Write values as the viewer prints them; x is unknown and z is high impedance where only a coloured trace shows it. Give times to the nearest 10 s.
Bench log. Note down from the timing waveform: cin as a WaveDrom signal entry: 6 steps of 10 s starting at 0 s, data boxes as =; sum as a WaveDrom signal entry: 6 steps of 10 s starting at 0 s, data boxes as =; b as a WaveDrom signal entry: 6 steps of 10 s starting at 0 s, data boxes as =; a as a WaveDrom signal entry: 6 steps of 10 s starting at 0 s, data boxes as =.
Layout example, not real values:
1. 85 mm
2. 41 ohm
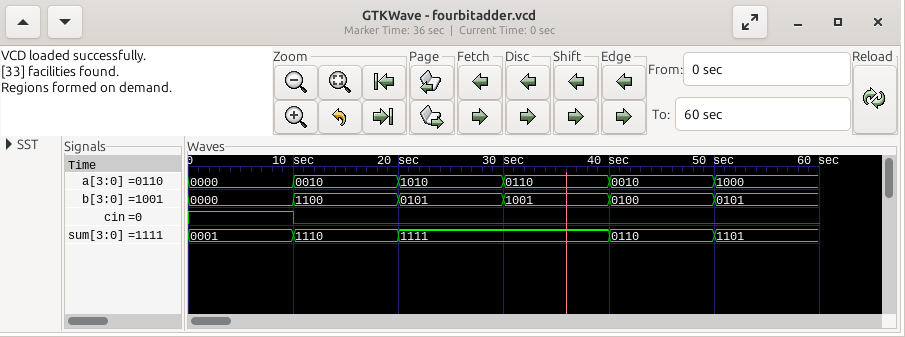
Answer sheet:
1. {name: 'cin', wave: '10....'}
2. {name: 'sum', wave: '===.==', data: '0001 1110 1111 0110 1101'}
3. {name: 'b', wave: '======', data: '0000 1100 0101 1001 0100 0101'}
4. {name: 'a', wave: '======', data: '0000 0010 1010 0110 0010 1000'}
